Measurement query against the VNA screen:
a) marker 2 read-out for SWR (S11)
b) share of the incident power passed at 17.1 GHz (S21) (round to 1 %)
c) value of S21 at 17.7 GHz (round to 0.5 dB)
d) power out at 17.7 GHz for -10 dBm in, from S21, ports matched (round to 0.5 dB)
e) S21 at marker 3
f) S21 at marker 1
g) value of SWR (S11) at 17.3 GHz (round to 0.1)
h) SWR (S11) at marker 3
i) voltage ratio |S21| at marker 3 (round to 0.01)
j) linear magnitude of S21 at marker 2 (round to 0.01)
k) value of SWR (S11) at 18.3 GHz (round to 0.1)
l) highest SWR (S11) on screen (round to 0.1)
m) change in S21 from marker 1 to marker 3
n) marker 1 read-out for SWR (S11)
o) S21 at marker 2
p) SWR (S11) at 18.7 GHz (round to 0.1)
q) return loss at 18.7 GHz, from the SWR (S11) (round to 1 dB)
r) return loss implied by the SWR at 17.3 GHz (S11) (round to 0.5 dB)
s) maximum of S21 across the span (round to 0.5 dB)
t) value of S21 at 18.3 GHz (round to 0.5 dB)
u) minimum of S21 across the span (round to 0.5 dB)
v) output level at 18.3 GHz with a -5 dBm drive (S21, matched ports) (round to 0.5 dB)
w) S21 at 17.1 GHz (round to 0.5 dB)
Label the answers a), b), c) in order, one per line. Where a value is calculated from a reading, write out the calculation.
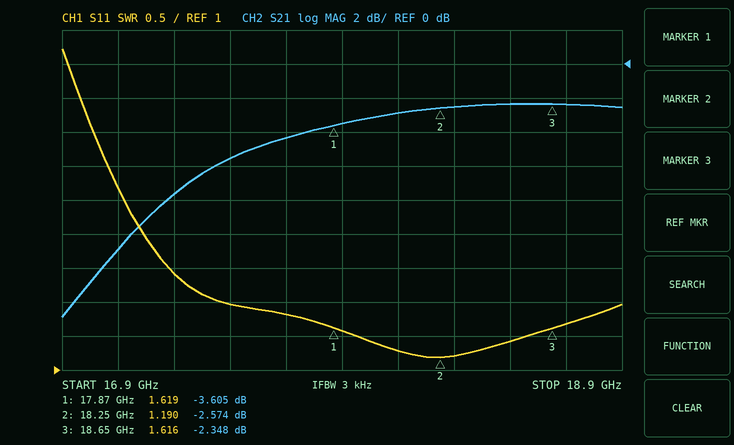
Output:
a) 1.190
b) 10^(-11/10) ≈ 8 %
c) -4.5 dB
d) -10 dBm + (-4.5 dB) = -14.5 dBm
e) -2.348 dB
f) -3.605 dB
g) 2.4
h) 1.616
i) 10^(-2.348/20) ≈ 0.76
j) 10^(-2.574/20) ≈ 0.74
k) 1.2
l) 5.7
m) -2.348 − (-3.605) = 1.257 dB
n) 1.619
o) -2.574 dB
p) 1.7
q) −20 log10((1.7 − 1)/(1.7 + 1)) ≈ 12 dB
r) −20 log10((2.4 − 1)/(2.4 + 1)) ≈ 7.71 dB, so 7.5 dB to the nearest 0.5 dB
s) -2.5 dB
t) -2.5 dB
u) -15.0 dB
v) -5 dBm + (-2.5 dB) = -7.5 dBm
w) -11.0 dB
